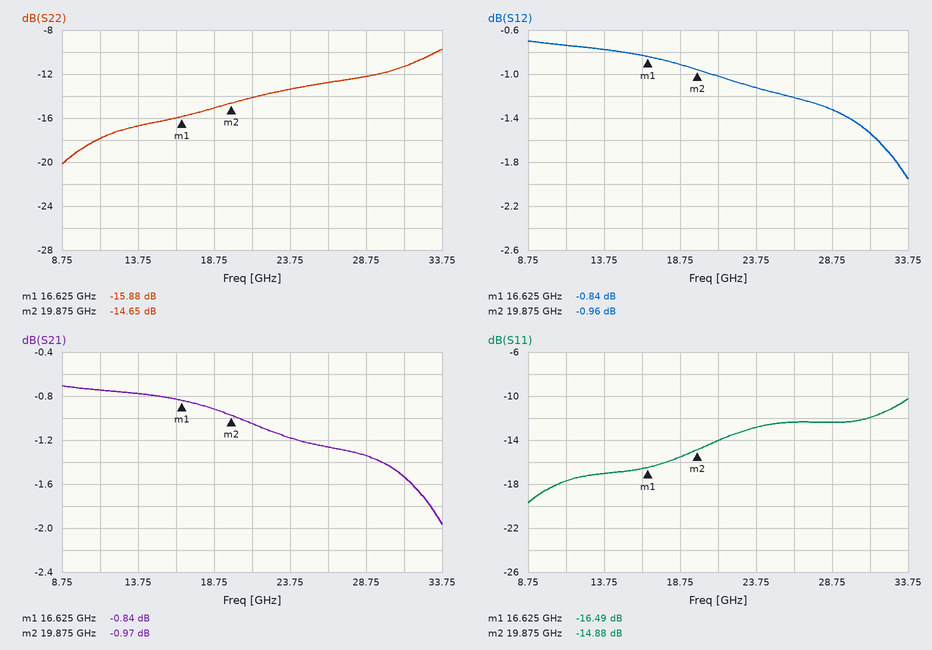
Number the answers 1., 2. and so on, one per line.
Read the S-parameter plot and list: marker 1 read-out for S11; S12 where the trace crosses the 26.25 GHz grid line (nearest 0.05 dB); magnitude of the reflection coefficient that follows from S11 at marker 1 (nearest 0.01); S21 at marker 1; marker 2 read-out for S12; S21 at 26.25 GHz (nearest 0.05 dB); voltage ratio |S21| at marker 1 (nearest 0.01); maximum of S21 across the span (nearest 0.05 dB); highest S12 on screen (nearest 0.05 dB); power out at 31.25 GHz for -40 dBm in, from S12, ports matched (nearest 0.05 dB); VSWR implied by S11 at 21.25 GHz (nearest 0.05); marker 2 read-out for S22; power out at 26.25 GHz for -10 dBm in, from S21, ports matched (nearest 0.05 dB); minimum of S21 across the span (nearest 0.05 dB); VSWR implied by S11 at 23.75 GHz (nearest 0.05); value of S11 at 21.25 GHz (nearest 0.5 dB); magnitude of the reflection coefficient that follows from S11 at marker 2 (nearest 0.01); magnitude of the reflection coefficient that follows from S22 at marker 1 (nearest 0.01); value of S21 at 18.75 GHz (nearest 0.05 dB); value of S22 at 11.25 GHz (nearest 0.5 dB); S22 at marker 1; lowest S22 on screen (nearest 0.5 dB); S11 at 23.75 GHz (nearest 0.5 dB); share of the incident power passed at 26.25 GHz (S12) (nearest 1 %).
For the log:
1. -16.49 dB
2. -1.20 dB
3. 0.15
4. -0.84 dB
5. -0.96 dB
6. -1.25 dB
7. 0.91
8. -0.70 dB
9. -0.70 dB
10. -41.55 dBm
11. 1.50
12. -14.65 dB
13. -11.25 dBm
14. -1.95 dB
15. 1.60
16. -14.0 dB
17. 0.18
18. 0.16
19. -0.90 dB
20. -18.0 dB
21. -15.88 dB
22. -20.0 dB
23. -13.0 dB
24. 76 %
